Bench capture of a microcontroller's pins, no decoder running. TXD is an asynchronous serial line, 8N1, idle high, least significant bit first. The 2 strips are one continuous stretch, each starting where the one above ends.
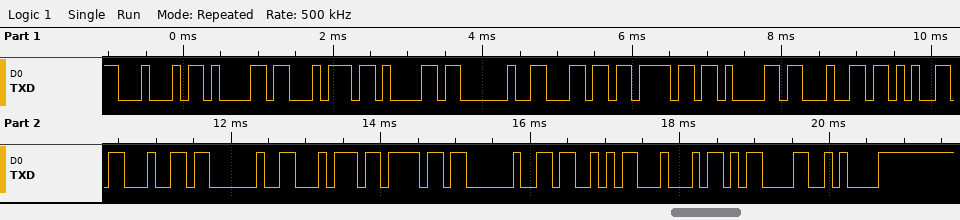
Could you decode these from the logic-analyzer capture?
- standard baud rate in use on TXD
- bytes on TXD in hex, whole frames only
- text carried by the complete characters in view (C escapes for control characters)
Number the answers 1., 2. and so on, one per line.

1. 9600 baud
2. 44 61 74 61 20 6C 6F 61 64 65 64 20 74 6F 20 53 44 0D 0A
3. "Data loaded to SD\r\n"
